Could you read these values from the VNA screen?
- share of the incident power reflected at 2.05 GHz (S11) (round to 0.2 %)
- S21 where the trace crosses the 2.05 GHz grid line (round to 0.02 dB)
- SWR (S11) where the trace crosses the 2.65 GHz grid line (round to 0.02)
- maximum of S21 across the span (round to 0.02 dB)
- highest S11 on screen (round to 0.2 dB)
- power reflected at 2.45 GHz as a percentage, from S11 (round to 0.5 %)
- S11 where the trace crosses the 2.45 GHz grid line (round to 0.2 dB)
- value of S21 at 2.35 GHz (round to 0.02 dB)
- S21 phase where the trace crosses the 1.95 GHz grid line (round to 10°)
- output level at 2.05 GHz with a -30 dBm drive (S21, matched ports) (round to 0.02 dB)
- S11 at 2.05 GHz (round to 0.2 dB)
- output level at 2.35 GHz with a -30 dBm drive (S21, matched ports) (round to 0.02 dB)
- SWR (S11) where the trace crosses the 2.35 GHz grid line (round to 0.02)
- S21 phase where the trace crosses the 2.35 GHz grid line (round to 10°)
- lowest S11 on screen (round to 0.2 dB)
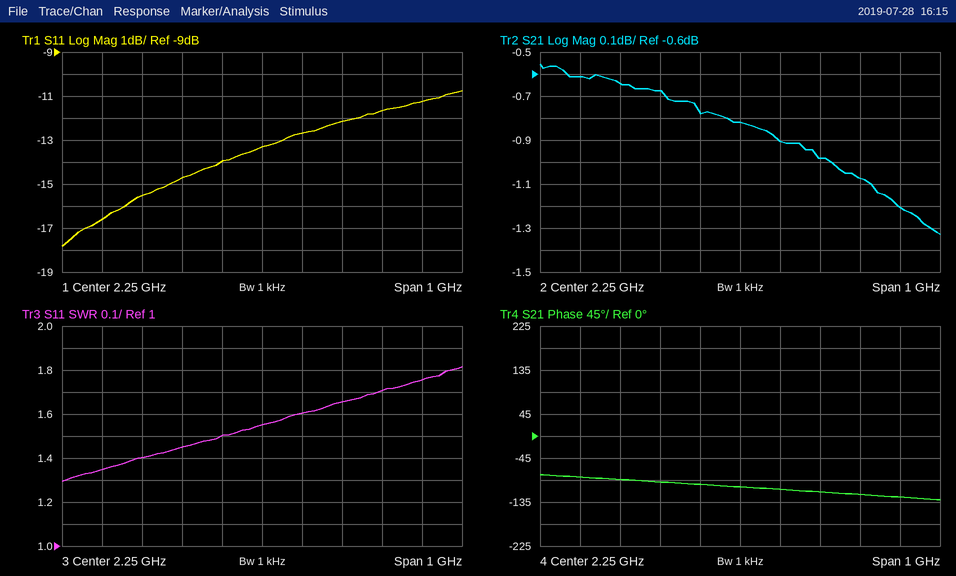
3.4 %
-0.68 dB
1.76
-0.56 dB
-10.8 dB
6.0 %
-12.2 dB
-0.90 dB
-90°
-30.68 dBm
-14.8 dB
-30.90 dBm
1.60
-110°
-17.8 dB
